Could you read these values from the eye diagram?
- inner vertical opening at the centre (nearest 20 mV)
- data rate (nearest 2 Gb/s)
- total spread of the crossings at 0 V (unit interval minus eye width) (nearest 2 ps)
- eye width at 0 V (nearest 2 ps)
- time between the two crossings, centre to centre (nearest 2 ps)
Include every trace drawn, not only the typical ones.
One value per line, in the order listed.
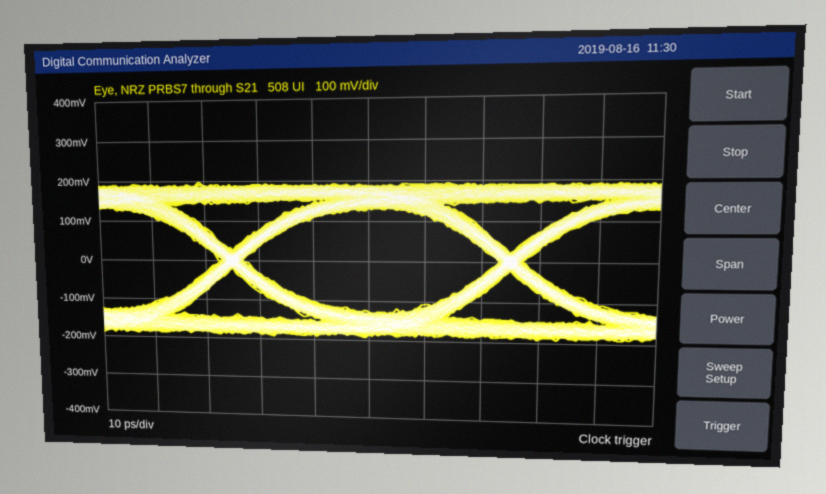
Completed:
260 mV
20 Gb/s
4 ps
46 ps
50 ps
